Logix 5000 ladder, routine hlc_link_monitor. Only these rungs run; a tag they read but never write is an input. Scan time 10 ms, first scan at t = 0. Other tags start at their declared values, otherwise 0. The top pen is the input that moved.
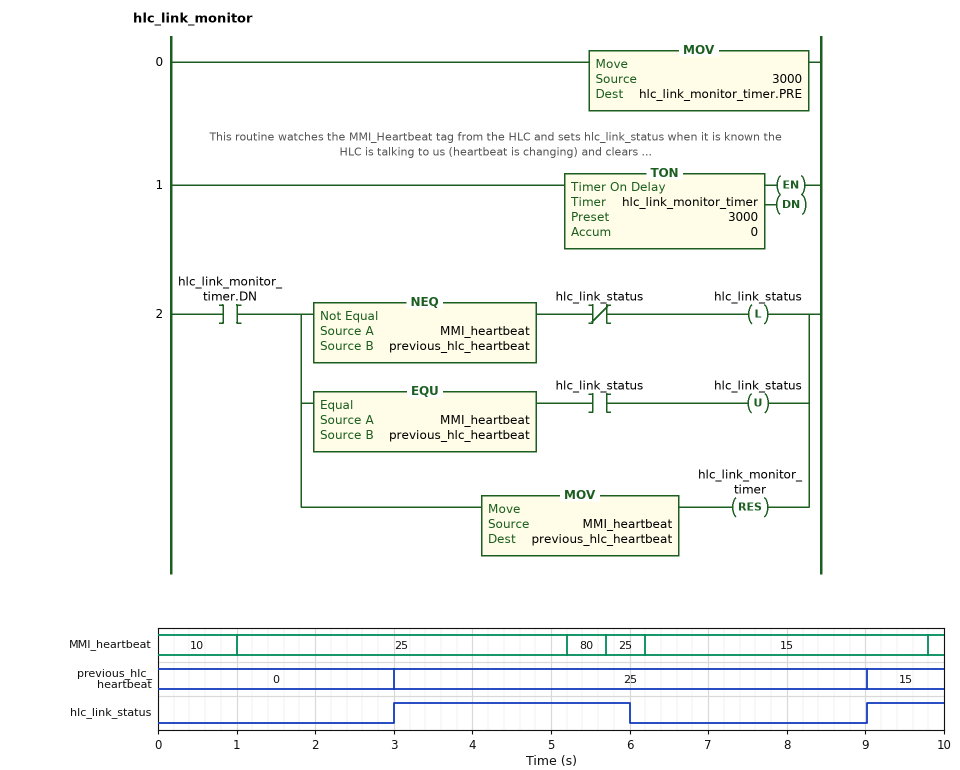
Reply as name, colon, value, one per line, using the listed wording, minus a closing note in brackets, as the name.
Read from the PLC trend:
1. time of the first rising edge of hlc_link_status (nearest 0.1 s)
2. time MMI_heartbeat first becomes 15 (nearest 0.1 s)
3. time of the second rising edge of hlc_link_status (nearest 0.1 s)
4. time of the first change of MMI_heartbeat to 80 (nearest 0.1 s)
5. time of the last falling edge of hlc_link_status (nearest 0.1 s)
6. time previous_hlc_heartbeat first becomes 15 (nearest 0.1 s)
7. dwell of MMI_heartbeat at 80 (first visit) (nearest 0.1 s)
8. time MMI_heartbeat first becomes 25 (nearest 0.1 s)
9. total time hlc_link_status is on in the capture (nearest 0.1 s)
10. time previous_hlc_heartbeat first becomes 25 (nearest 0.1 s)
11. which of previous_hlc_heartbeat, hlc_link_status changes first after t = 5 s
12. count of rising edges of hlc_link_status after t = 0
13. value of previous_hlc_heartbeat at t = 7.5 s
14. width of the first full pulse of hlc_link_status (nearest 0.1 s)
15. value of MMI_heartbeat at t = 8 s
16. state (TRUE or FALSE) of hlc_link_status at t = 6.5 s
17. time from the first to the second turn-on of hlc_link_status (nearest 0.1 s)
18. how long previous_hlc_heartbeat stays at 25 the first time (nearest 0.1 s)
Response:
time of the first rising edge of hlc_link_status: 3.0 s
time MMI_heartbeat first becomes 15: 6.2 s
time of the second rising edge of hlc_link_status: 9.0 s
time of the first change of MMI_heartbeat to 80: 5.2 s
time of the last falling edge of hlc_link_status: 6.0 s
time previous_hlc_heartbeat first becomes 15: 9.0 s
dwell of MMI_heartbeat at 80 (first visit): 0.5 s
time MMI_heartbeat first becomes 25: 1.0 s
total time hlc_link_status is on in the capture: 4.0 s
time previous_hlc_heartbeat first becomes 25: 3.0 s
which of previous_hlc_heartbeat, hlc_link_status changes first after t = 5 s: hlc_link_status
count of rising edges of hlc_link_status after t = 0: 2
value of previous_hlc_heartbeat at t = 7.5 s: 25
width of the first full pulse of hlc_link_status: 3.0 s
value of MMI_heartbeat at t = 8 s: 15
state (TRUE or FALSE) of hlc_link_status at t = 6.5 s: FALSE
time from the first to the second turn-on of hlc_link_status: 6.0 s
how long previous_hlc_heartbeat stays at 25 the first time: 6.0 s
